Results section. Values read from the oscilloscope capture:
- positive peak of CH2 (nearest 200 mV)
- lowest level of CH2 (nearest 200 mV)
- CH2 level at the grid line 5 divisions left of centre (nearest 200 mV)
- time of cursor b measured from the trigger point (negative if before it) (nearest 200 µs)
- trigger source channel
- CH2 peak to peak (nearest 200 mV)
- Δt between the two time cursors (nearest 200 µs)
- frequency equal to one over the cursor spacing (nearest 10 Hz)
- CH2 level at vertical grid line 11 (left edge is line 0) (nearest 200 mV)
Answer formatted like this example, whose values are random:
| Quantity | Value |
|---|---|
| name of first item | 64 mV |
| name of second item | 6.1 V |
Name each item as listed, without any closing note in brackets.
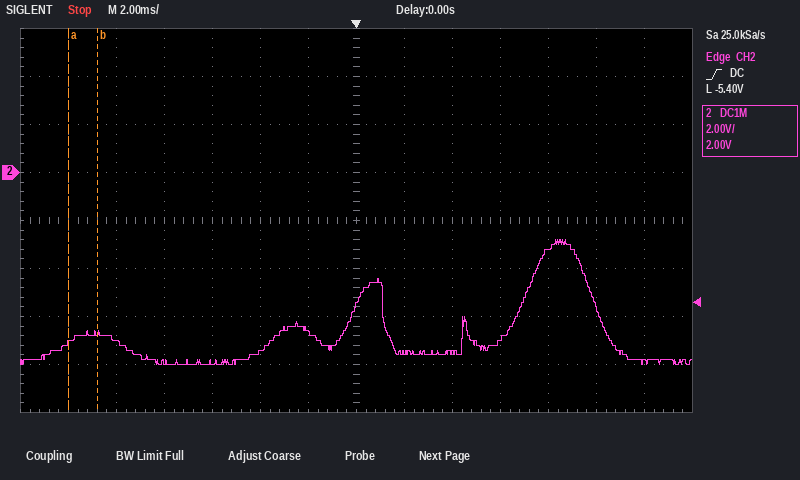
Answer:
| Quantity | Value |
|---|---|
| positive peak of CH2 | -2.8 V |
| lowest level of CH2 | -8.0 V |
| CH2 level at the grid line 5 divisions left of centre | -7.0 V |
| time of cursor b measured from the trigger point (negative if before it) | -10.8 ms |
| trigger source channel | CH2 |
| CH2 peak to peak | 5.2 V |
| Δt between the two time cursors | 1.2 ms |
| frequency equal to one over the cursor spacing | 830 Hz |
| CH2 level at vertical grid line 11 (left edge is line 0) | -3.2 V |
